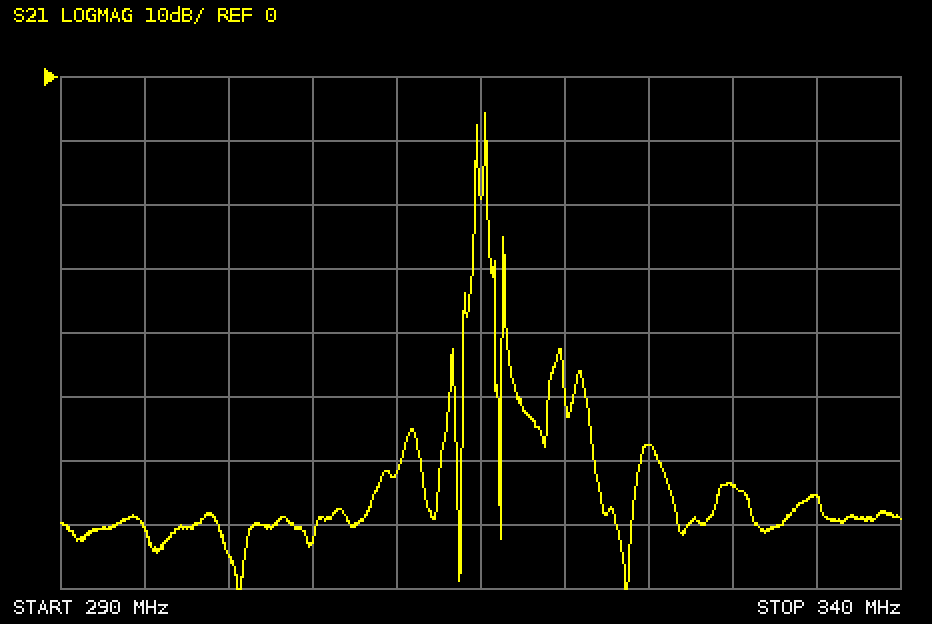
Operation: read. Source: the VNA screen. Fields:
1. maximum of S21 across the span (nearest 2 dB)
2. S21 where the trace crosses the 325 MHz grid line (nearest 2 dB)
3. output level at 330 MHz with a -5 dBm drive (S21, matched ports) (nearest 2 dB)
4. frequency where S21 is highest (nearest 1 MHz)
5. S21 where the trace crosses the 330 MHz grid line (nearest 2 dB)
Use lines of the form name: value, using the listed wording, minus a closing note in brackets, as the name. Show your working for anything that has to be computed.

maximum of S21 across the span: -6 dB
S21 where the trace crosses the 325 MHz grid line: -58 dB
output level at 330 MHz with a -5 dBm drive (S21, matched ports): -5 dBm + (-64 dB) = -68 dBm
frequency where S21 is highest: 315 MHz
S21 where the trace crosses the 330 MHz grid line: -64 dB
